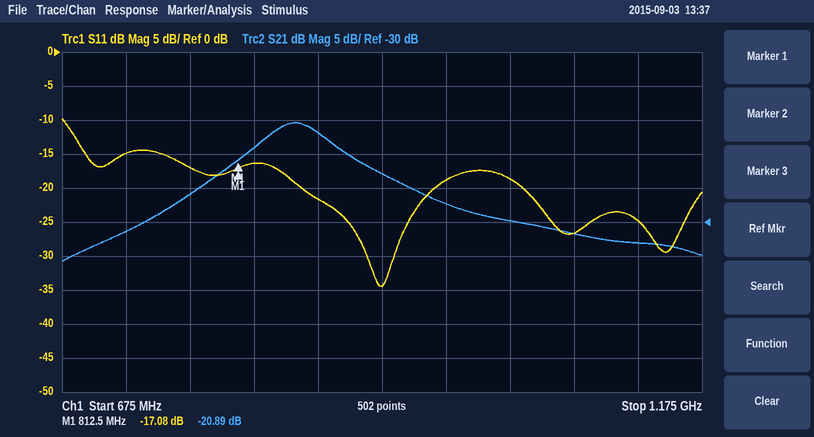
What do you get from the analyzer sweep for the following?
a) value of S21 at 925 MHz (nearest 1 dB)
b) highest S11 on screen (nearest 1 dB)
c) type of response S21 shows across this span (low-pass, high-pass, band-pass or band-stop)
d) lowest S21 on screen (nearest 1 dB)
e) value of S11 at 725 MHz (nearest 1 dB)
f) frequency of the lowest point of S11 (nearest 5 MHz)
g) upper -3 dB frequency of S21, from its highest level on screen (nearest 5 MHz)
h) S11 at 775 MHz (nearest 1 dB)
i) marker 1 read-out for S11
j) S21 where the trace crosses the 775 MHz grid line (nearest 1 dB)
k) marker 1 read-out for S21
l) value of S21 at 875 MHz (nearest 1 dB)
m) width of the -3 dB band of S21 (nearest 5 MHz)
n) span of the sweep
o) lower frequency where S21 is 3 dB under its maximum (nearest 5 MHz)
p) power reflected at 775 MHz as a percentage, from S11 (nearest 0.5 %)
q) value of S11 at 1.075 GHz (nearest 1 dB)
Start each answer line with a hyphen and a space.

- -23 dB
- -10 dB
- band-pass
- -36 dB
- -15 dB
- 925 MHz
- 885 MHz
- -17 dB
- -17.08 dB
- -26 dB
- -20.89 dB
- -17 dB
- 55 MHz
- 500 MHz
- 830 MHz
- 2.0 %
- -27 dB
